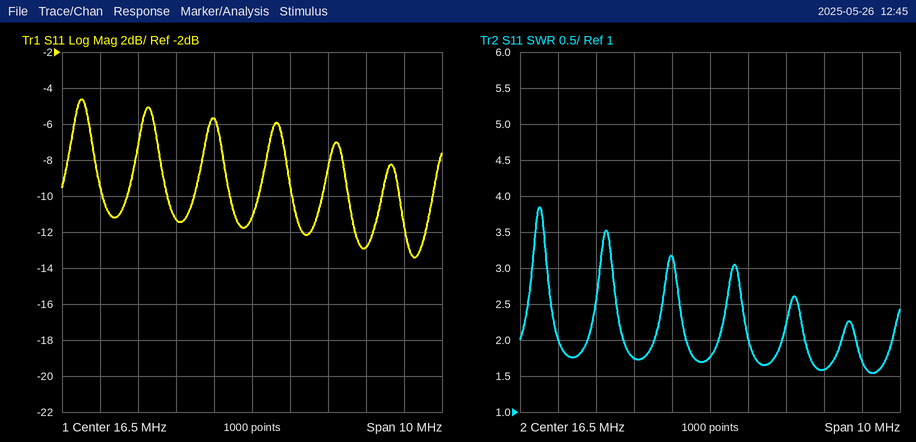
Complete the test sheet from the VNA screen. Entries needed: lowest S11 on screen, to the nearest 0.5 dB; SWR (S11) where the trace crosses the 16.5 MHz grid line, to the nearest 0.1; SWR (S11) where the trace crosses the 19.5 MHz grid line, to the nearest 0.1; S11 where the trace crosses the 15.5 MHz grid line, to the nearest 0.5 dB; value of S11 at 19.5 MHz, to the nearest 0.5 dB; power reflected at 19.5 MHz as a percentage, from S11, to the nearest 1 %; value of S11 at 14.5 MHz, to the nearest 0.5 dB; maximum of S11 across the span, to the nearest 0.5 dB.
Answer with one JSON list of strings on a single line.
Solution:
["-13.5 dB", "1.8", "1.6", "-5.5 dB", "-13.0 dB", "5 %", "-11.5 dB", "-4.5 dB"]
